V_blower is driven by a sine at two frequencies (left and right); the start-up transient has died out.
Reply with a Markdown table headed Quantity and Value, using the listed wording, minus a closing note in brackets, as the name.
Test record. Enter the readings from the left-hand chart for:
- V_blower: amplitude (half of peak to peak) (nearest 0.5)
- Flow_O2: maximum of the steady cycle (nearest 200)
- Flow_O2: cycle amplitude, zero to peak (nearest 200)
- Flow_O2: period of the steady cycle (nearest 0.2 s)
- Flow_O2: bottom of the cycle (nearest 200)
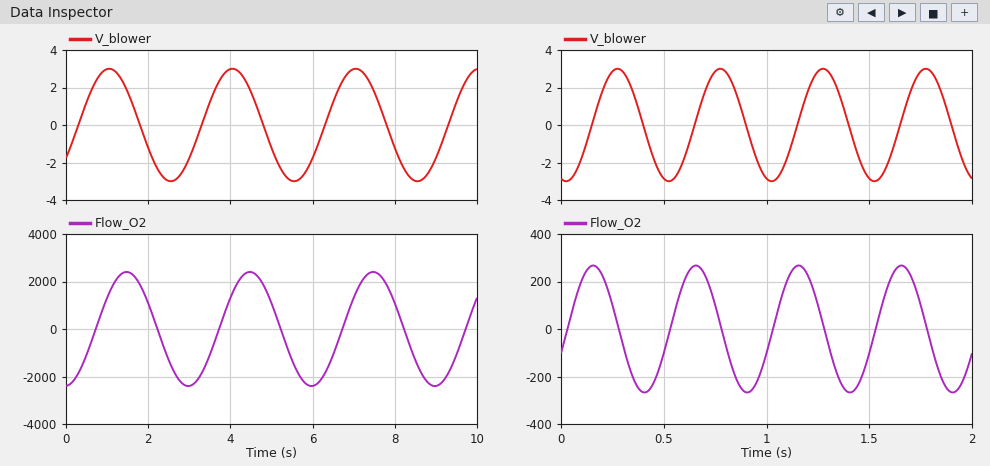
| Quantity | Value |
|---|---|
| V_blower: amplitude (half of peak to peak) | 3.0 |
| Flow_O2: maximum of the steady cycle | 2400 |
| Flow_O2: cycle amplitude, zero to peak | 2400 |
| Flow_O2: period of the steady cycle | 3.0 s |
| Flow_O2: bottom of the cycle | -2400 |
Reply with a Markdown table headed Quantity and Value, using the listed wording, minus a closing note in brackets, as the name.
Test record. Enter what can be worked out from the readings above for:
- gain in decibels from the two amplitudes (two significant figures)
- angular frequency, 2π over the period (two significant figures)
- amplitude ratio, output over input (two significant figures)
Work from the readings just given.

| Quantity | Value |
|---|---|
| gain in decibels from the two amplitudes | 58 dB |
| angular frequency, 2π over the period | 2.1 rad/s |
| amplitude ratio, output over input | 800 |
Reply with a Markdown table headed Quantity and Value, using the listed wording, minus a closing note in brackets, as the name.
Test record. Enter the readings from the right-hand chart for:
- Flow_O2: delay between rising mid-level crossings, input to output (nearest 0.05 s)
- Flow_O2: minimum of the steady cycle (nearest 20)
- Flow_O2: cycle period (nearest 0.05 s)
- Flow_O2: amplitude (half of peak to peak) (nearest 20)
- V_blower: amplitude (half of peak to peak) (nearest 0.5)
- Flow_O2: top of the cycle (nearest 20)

| Quantity | Value |
|---|---|
| Flow_O2: delay between rising mid-level crossings, input to output | 0.40 s |
| Flow_O2: minimum of the steady cycle | -260 |
| Flow_O2: cycle period | 0.50 s |
| Flow_O2: amplitude (half of peak to peak) | 260 |
| V_blower: amplitude (half of peak to peak) | 3.0 |
| Flow_O2: top of the cycle | 260 |
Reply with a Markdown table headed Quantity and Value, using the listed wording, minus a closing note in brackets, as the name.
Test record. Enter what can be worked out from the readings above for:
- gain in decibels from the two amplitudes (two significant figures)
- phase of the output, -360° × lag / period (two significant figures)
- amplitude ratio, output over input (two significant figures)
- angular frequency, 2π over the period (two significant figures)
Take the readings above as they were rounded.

| Quantity | Value |
|---|---|
| gain in decibels from the two amplitudes | 39 dB |
| phase of the output, -360° × lag / period | -290° |
| amplitude ratio, output over input | 87 |
| angular frequency, 2π over the period | 13 rad/s |
